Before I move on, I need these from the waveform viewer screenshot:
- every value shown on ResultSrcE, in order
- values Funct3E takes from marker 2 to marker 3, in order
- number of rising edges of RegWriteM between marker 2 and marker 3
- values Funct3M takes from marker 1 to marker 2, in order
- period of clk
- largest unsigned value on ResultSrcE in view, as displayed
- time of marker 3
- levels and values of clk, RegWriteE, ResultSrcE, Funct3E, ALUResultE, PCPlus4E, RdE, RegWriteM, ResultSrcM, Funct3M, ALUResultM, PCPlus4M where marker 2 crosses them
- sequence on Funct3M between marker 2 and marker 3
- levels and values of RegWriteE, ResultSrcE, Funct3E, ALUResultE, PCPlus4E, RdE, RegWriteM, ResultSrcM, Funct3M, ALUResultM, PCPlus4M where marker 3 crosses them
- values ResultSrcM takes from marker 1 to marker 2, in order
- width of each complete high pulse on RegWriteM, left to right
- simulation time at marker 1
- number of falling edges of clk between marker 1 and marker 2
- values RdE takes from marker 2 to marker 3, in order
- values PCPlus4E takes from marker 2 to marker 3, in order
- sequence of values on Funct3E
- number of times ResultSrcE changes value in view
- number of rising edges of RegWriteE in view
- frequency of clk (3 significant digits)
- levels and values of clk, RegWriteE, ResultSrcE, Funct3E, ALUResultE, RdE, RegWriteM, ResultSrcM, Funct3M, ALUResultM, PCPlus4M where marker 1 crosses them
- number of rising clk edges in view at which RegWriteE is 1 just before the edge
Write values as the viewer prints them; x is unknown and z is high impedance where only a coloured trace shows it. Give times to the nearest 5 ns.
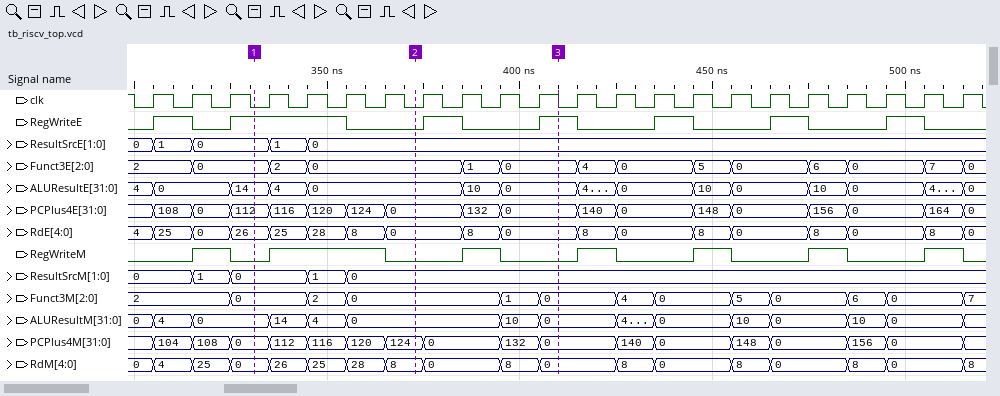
0, 1, 0, 1, 0
0, 1, 0
1
0, 2, 0
10 ns
1
410 ns
clk=0, RegWriteE=0, ResultSrcE=0, Funct3E=0, ALUResultE=0, PCPlus4E=0, RdE=0, RegWriteM=0, ResultSrcM=0, Funct3M=0, ALUResultM=0, PCPlus4M=124
0, 1, 0
RegWriteE=1, ResultSrcE=0, Funct3E=0, ALUResultE=0, PCPlus4E=0, RdE=0, RegWriteM=0, ResultSrcM=0, Funct3M=0, ALUResultM=0, PCPlus4M=0
0, 1, 0
10 ns, 30 ns, 10 ns, 10 ns, 10 ns, 10 ns, 10 ns
330 ns
4
0, 8, 0
0, 132, 0
2, 0, 2, 0, 1, 0, 4, 0, 5, 0, 6, 0, 7, 0
4
7
100 MHz
clk=0, RegWriteE=1, ResultSrcE=0, Funct3E=0, ALUResultE=14, RdE=26, RegWriteM=0, ResultSrcM=0, Funct3M=0, ALUResultM=0, PCPlus4M=0
9
